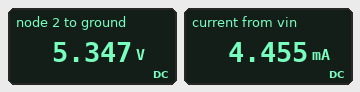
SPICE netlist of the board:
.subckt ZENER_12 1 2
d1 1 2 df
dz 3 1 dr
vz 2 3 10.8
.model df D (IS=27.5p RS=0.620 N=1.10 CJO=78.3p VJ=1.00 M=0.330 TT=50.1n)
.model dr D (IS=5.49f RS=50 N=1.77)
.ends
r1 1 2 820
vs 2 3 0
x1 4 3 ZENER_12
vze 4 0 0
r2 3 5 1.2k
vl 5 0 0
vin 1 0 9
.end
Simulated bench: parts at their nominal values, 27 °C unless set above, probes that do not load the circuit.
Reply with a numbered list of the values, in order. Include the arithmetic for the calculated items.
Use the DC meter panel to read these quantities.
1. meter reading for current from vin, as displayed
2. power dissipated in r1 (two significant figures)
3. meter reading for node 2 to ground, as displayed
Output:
1. 4.455 mA
2. (9 V - 5.347 V)^2 / 820 Ω = 16 mW
3. 5.347 V
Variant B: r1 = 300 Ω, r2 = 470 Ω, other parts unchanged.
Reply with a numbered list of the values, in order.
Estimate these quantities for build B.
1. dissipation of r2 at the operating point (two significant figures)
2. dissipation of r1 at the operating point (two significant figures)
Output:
1. 64 mW
2. 41 mW
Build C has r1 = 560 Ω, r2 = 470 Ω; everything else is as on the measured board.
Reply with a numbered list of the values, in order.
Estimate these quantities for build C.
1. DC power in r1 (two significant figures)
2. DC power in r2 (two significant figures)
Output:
1. 43 mW
2. 36 mW
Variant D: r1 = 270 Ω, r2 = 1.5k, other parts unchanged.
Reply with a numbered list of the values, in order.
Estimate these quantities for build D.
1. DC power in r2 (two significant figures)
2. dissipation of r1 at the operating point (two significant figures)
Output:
1. 39 mW
2. 7.0 mW
